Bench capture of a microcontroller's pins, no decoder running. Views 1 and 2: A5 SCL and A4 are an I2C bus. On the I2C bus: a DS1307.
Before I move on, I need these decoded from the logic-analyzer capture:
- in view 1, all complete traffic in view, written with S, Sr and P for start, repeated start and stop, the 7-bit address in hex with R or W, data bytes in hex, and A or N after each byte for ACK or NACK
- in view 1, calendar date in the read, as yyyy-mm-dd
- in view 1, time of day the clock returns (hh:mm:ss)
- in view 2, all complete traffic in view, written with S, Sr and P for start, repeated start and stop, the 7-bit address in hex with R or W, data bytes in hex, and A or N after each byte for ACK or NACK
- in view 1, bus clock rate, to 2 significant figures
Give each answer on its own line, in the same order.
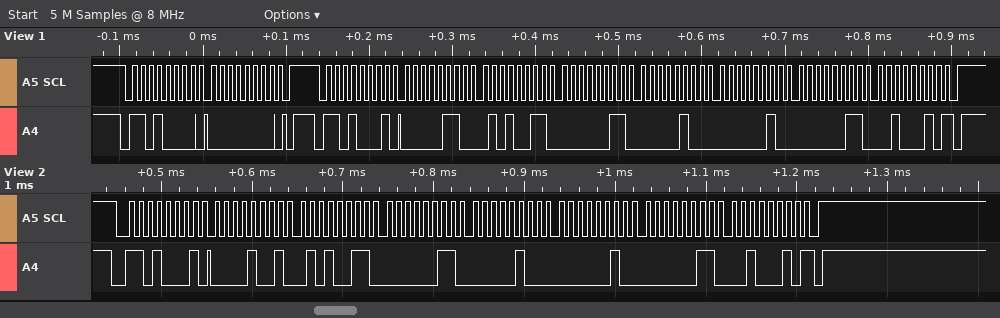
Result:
S 68W A 00 A P S 68R A 06 A 53 A 03 A 04 A 02 A 03 A 22 N P
2022-03-02
03:53:06
S 68R A 09 A 53 A 03 A 04 A 02 A 03 A 22 N P
100 kHz
